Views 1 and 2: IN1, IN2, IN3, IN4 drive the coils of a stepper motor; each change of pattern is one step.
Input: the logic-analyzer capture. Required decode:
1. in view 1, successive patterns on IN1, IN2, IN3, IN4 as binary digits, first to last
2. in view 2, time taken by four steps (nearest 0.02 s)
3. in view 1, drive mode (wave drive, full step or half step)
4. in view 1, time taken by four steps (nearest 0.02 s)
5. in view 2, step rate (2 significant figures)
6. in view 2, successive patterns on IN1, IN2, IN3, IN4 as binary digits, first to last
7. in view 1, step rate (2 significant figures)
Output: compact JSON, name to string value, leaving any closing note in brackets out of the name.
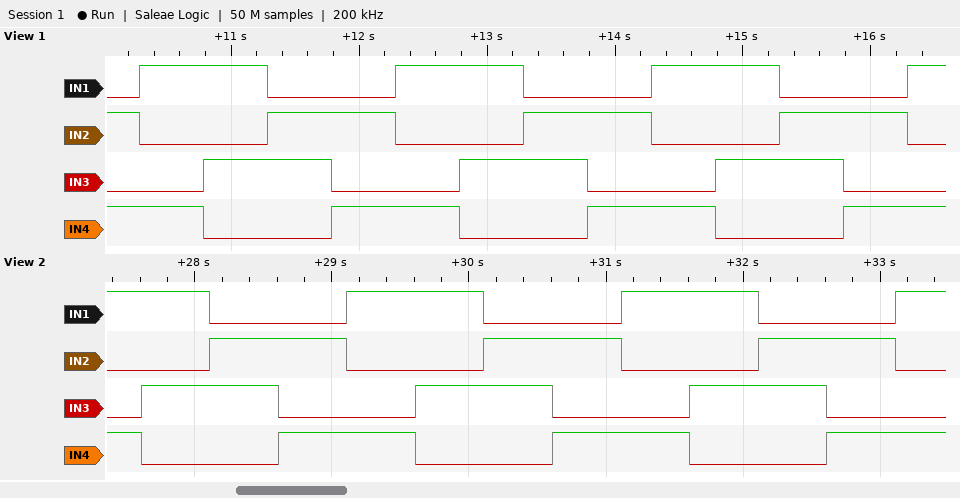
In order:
{"in view 1, successive patterns on IN1, IN2, IN3, IN4 as binary digits, first to last": "0101 1001 1010 0110 0101 1001 1010 0110 0101 1001 1010 0110 0101 1001", "in view 2, time taken by four steps": "2.00 s", "in view 1, drive mode": "full step", "in view 1, time taken by four steps": "2.00 s", "in view 2, step rate": "2.0 steps/s", "in view 2, successive patterns on IN1, IN2, IN3, IN4 as binary digits, first to last": "1001 1010 0110 0101 1001 1010 0110 0101 1001 1010 0110 0101 1001", "in view 1, step rate": "2.0 steps/s"}
